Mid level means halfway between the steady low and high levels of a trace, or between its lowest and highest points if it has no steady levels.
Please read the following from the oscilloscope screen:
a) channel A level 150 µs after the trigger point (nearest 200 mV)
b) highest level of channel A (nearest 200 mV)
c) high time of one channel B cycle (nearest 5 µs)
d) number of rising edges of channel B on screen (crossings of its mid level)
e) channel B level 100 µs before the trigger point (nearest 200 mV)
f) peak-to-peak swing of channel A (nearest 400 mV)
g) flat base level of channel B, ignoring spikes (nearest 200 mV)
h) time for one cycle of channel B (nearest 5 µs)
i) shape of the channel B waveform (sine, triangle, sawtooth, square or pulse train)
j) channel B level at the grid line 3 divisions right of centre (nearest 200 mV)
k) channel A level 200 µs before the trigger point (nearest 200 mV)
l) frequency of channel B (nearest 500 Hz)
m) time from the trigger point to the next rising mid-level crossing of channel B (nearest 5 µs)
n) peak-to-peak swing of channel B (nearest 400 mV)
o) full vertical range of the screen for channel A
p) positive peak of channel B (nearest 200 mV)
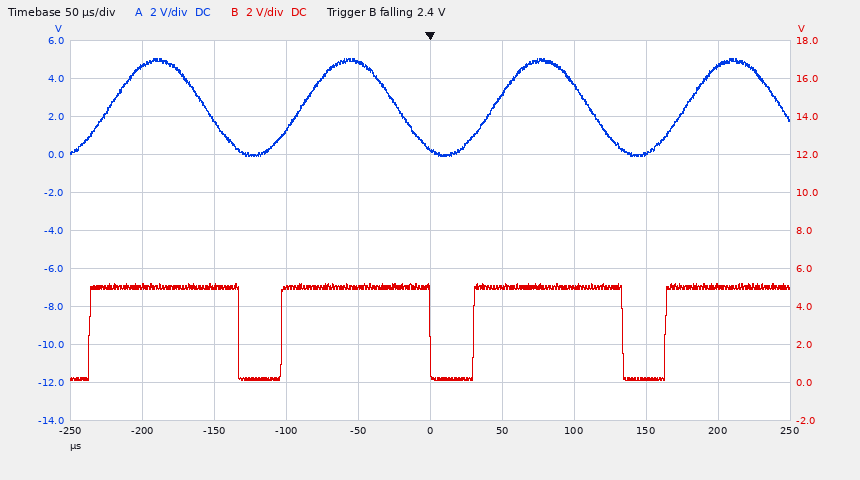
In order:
0.0 V
5.0 V
105 µs
4
5.0 V
5.2 V
200 mV
135 µs
pulse train
200 mV
4.6 V
7.5 kHz
30 µs
5.2 V
20 V
5.2 V
